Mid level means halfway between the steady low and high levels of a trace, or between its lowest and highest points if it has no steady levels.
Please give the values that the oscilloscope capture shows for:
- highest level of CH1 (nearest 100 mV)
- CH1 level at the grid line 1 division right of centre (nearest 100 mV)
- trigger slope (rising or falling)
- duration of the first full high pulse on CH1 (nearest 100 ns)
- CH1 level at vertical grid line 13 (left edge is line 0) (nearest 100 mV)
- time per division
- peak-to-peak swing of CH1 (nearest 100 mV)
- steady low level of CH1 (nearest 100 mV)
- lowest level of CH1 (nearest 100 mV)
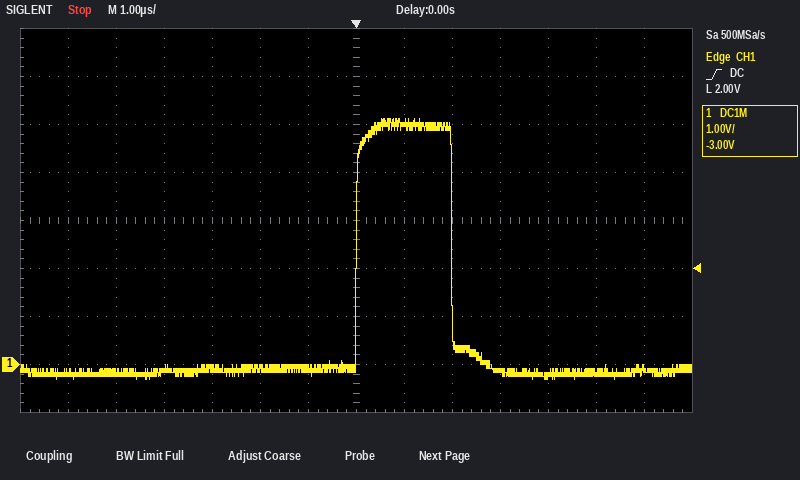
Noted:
5.1 V
5.0 V
rising
2.0 µs
-100 mV
1 µs
5.4 V
-200 mV
-300 mV
